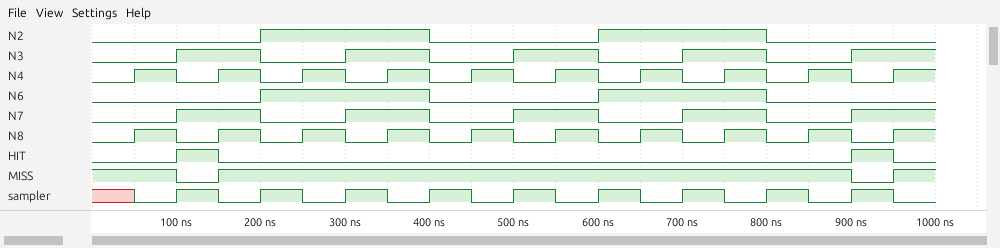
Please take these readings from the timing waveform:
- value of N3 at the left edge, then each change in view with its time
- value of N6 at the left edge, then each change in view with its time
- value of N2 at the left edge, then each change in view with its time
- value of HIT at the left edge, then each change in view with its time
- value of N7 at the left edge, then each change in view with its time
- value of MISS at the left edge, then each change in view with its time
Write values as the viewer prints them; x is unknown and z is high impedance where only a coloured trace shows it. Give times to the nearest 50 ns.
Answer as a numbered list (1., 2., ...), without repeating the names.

1. 0, 1 at 100 ns, 0 at 200 ns, 1 at 300 ns, 0 at 400 ns, 1 at 500 ns, 0 at 600 ns, 1 at 700 ns, 0 at 800 ns, 1 at 900 ns
2. 0, 1 at 200 ns, 0 at 400 ns, 1 at 600 ns, 0 at 800 ns
3. 0, 1 at 200 ns, 0 at 400 ns, 1 at 600 ns, 0 at 800 ns
4. 0, 1 at 100 ns, 0 at 150 ns, 1 at 900 ns, 0 at 950 ns
5. 0, 1 at 100 ns, 0 at 200 ns, 1 at 300 ns, 0 at 400 ns, 1 at 500 ns, 0 at 600 ns, 1 at 700 ns, 0 at 800 ns, 1 at 900 ns
6. 1, 0 at 100 ns, 1 at 150 ns, 0 at 900 ns, 1 at 950 ns
